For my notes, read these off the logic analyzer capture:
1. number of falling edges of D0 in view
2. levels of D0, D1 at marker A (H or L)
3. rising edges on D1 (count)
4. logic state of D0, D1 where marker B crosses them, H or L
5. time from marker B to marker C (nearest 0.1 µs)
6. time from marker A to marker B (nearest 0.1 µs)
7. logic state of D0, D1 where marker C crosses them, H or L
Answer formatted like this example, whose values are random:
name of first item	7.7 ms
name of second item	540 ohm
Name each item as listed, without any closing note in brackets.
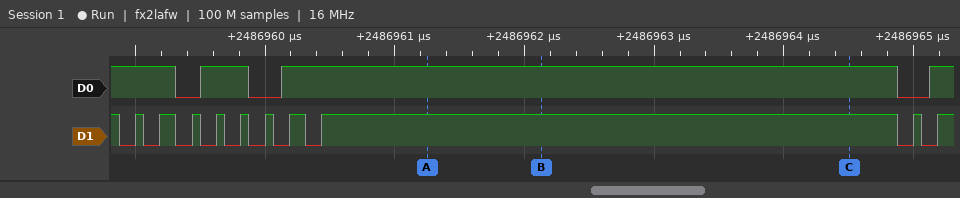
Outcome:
number of falling edges of D0 in view	3
levels of D0, D1 at marker A	D0=H, D1=H
rising edges on D1	10
logic state of D0, D1 where marker B crosses them, H or L	D0=H, D1=H
time from marker B to marker C	2.4 µs
time from marker A to marker B	0.9 µs
logic state of D0, D1 where marker C crosses them, H or L	D0=H, D1=H
